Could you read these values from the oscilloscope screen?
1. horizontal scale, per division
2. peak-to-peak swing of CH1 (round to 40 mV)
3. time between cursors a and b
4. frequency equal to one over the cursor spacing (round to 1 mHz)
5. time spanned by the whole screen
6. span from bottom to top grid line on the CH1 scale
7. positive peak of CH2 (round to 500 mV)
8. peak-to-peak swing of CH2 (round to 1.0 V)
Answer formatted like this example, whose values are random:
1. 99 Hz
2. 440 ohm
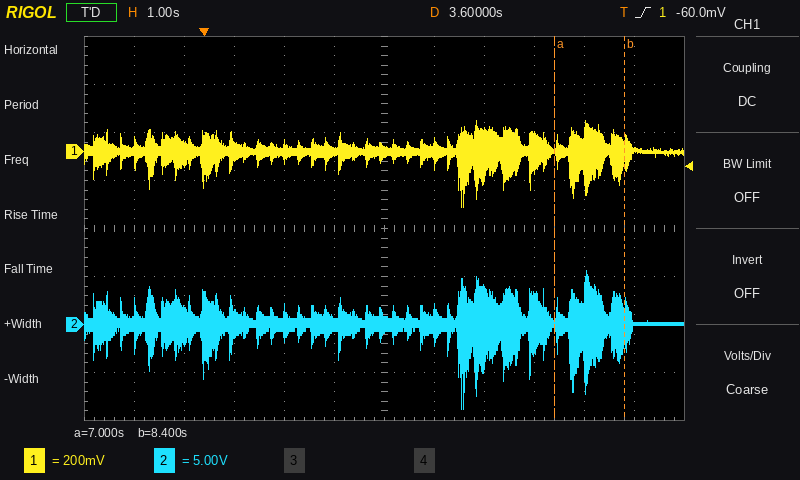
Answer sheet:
1. 1 s
2. 360 mV
3. 1.4 s
4. 714 mHz
5. 12 s
6. 1.6 V
7. 5.5 V
8. 14.0 V
